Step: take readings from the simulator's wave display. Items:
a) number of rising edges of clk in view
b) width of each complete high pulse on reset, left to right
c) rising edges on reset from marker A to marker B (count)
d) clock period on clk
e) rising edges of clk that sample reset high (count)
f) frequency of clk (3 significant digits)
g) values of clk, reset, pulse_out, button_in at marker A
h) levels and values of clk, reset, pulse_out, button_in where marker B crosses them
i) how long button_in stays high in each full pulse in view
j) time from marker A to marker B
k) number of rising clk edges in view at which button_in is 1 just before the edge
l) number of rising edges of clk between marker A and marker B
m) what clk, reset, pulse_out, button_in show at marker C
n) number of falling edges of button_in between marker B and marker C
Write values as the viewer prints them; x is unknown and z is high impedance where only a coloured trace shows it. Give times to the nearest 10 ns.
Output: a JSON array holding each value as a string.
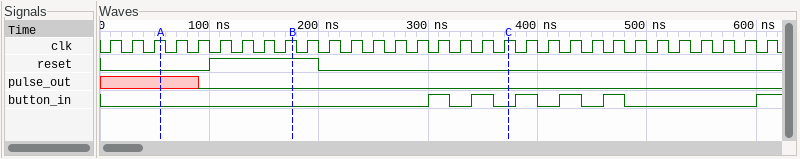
["31", "100 ns", "1", "20 ns", "5", "50.0 MHz", "clk=1, reset=0, pulse_out=x, button_in=0", "clk=1, reset=1, pulse_out=0, button_in=0", "20 ns, 20 ns, 20 ns, 20 ns, 20 ns", "120 ns", "6", "6", "clk=1, reset=0, pulse_out=0, button_in=0", "2"]
